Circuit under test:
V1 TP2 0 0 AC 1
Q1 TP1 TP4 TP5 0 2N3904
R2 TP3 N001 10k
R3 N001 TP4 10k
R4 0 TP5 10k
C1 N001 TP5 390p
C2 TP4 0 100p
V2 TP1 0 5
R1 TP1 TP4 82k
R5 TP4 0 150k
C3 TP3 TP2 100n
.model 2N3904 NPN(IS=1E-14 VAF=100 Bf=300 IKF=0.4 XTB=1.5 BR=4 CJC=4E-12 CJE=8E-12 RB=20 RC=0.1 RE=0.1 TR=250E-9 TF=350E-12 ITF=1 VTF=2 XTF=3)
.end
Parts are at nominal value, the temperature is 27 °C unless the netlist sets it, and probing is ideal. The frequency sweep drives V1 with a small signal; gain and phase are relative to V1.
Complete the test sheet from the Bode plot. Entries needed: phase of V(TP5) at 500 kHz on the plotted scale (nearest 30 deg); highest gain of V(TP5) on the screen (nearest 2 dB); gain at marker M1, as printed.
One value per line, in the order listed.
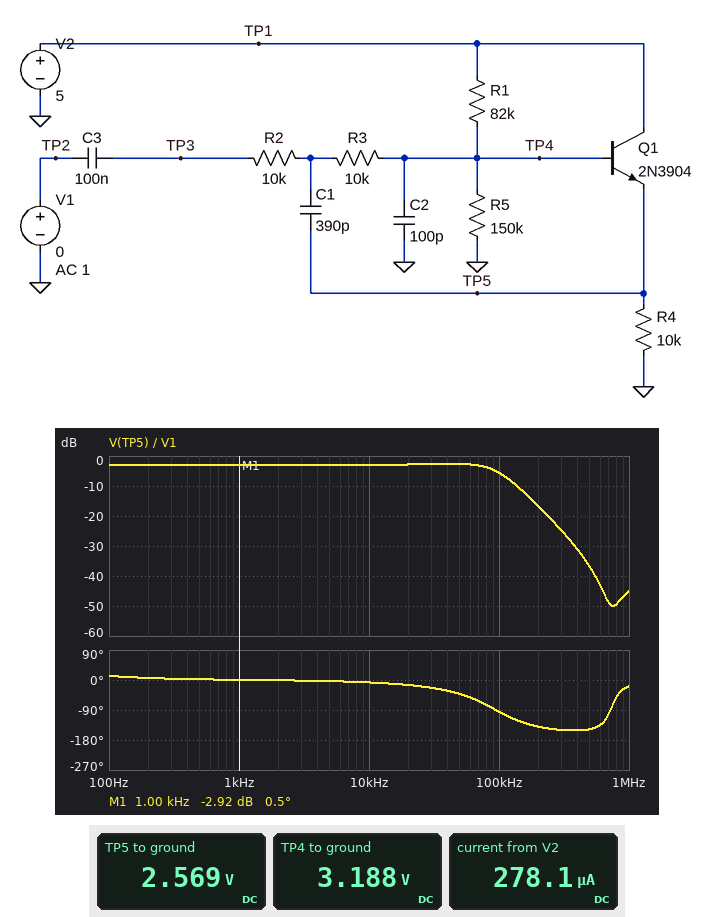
-150 deg
-2 dB
-2.92 dB
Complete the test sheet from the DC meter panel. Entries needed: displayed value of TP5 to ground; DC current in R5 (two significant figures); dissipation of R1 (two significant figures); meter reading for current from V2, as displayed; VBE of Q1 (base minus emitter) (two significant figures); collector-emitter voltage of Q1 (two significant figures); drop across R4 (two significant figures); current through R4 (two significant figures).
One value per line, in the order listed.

2.569 V
21 µA
40 µW
278.1 µA
620 mV
2.4 V
2.6 V
260 µA
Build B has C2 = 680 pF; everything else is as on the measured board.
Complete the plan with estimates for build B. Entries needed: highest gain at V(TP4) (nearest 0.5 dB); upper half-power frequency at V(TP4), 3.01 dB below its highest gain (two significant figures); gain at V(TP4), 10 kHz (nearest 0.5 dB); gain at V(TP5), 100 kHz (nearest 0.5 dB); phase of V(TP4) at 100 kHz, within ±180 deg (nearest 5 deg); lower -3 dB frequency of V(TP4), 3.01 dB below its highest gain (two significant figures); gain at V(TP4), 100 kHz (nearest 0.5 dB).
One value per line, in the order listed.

-3.0 dB
18 kHz
-4.0 dB
-23.5 dB
-135 deg
22 Hz
-22.5 dB
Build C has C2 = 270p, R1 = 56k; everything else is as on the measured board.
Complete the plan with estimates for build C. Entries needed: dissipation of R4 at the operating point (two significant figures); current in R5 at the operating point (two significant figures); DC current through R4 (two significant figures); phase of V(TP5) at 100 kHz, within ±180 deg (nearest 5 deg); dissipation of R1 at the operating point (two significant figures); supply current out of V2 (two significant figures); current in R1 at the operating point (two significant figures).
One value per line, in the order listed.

890 µW
24 µA
300 µA
-120 deg
35 µW
320 µA
25 µA
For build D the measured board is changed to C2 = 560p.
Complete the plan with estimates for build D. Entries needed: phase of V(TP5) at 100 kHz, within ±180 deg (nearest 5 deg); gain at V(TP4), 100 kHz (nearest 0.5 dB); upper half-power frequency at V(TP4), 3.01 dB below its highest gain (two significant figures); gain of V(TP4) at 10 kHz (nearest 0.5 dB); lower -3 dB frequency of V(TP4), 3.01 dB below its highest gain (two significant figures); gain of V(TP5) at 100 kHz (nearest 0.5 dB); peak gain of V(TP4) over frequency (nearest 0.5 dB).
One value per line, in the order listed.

-130 deg
-20.5 dB
23 kHz
-3.5 dB
22 Hz
-21.5 dB
-3.0 dB
